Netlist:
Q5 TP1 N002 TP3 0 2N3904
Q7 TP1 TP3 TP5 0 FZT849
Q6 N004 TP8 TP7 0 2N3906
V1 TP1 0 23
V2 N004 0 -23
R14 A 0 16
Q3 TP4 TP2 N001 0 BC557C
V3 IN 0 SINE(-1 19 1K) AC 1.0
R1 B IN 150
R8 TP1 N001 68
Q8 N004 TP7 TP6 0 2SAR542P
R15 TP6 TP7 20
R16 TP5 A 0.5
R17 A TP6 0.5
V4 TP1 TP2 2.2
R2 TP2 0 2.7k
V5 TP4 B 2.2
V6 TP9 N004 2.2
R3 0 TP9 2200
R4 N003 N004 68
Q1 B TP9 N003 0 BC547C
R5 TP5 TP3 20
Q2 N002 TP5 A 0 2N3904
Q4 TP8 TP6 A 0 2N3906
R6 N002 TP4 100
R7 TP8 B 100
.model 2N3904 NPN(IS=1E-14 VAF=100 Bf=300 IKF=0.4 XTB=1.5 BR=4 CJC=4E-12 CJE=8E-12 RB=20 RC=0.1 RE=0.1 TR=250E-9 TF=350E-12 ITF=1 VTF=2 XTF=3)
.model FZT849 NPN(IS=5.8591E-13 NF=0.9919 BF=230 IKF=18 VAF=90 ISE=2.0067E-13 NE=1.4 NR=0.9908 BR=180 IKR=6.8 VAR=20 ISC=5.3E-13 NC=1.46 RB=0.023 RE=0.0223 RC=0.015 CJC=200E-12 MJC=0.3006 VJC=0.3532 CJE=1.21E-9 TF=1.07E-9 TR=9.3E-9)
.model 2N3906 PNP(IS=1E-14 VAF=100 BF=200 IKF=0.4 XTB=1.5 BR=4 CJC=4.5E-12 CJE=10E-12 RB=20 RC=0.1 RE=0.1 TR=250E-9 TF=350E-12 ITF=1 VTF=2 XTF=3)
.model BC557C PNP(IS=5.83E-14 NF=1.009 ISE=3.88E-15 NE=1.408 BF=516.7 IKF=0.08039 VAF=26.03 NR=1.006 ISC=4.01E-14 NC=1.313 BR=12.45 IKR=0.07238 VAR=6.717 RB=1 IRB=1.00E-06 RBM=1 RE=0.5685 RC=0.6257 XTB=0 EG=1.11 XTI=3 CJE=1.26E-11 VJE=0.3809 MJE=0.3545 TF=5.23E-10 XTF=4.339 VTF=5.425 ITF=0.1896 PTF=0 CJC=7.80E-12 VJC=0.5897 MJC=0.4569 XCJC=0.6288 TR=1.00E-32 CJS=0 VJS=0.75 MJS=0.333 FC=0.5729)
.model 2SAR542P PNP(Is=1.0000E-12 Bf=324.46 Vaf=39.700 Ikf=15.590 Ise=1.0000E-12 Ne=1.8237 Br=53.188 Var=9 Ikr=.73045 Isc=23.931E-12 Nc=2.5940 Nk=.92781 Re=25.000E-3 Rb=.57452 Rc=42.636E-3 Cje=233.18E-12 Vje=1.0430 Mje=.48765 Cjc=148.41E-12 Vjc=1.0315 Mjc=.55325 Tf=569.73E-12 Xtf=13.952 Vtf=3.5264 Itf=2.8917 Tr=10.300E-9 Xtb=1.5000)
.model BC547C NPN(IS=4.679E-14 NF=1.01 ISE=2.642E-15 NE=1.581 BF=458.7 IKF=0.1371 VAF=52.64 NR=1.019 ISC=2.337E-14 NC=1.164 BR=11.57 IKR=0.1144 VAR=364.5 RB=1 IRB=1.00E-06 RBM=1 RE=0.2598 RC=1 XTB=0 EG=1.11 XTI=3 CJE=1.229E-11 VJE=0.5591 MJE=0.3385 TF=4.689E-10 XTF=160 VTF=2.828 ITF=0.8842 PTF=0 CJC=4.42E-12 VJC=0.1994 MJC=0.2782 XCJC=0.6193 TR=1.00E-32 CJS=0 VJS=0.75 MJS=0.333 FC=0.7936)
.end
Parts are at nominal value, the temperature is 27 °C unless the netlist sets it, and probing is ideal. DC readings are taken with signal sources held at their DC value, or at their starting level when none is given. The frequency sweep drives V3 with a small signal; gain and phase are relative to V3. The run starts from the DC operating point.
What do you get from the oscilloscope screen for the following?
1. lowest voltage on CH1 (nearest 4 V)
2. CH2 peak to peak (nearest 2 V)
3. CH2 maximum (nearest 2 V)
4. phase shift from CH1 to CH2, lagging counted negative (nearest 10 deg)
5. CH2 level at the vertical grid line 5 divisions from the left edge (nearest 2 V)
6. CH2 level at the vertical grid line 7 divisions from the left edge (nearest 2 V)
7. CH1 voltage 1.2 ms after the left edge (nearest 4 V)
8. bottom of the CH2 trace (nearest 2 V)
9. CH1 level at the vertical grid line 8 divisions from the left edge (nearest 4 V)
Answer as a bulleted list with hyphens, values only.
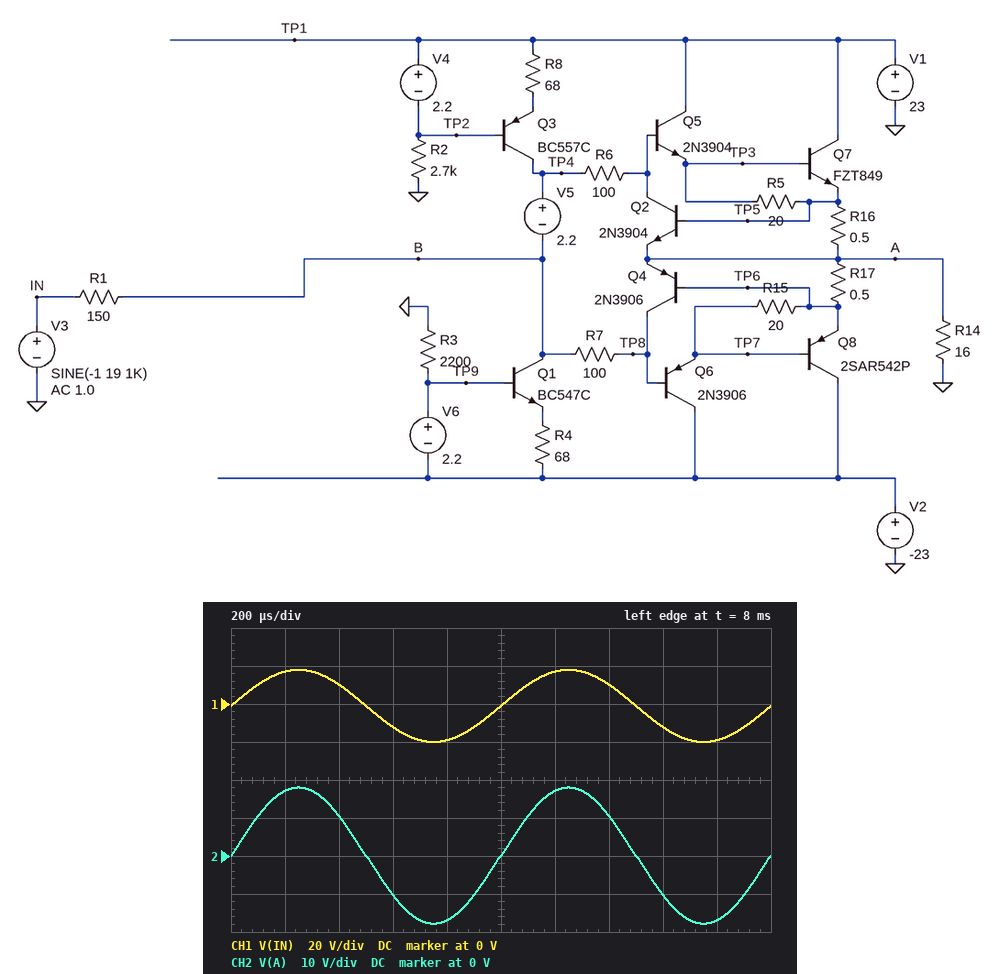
- -20 V
- 36 V
- 18 V
- 0 deg
- 0 V
- 10 V
- 16 V
- -18 V
- -12 V
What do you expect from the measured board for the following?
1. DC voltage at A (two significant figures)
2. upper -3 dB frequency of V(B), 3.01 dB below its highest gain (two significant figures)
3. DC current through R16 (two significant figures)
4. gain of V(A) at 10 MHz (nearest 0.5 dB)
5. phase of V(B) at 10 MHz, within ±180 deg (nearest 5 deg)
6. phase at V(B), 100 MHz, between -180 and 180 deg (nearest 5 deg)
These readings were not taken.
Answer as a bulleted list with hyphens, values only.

- 65 mV
- 36 MHz
- 20 mA
- -3.0 dB
- -15 deg
- -40 deg
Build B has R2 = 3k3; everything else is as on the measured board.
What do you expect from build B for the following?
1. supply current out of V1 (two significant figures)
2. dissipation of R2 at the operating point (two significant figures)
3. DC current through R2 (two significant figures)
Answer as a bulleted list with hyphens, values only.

- 48 mA
- 130 mW
- 6.3 mA
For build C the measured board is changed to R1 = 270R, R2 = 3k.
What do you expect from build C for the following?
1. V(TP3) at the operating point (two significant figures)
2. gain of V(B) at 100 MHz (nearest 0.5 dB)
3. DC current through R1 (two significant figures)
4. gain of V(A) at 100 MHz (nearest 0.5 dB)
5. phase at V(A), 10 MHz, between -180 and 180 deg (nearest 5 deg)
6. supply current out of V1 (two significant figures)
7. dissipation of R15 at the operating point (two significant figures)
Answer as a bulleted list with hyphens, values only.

- 480 mV
- -15.0 dB
- 64 µA
- -17.0 dB
- -15 deg
- 49 mA
- 4.9 mW
